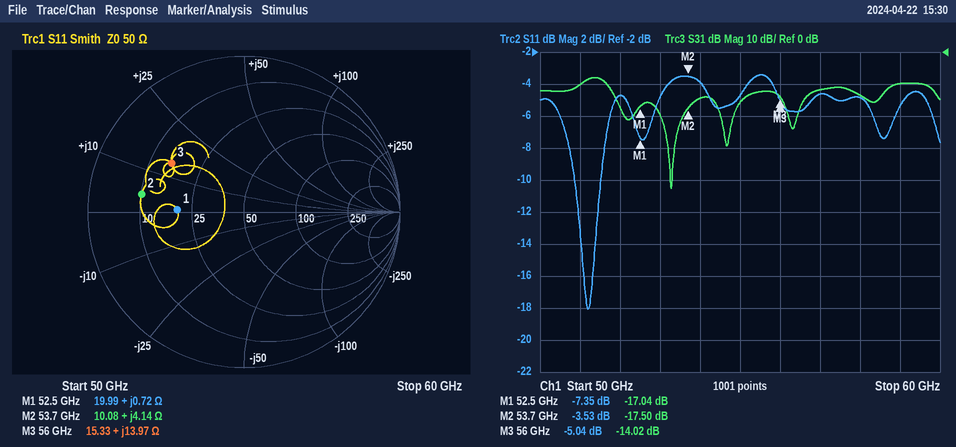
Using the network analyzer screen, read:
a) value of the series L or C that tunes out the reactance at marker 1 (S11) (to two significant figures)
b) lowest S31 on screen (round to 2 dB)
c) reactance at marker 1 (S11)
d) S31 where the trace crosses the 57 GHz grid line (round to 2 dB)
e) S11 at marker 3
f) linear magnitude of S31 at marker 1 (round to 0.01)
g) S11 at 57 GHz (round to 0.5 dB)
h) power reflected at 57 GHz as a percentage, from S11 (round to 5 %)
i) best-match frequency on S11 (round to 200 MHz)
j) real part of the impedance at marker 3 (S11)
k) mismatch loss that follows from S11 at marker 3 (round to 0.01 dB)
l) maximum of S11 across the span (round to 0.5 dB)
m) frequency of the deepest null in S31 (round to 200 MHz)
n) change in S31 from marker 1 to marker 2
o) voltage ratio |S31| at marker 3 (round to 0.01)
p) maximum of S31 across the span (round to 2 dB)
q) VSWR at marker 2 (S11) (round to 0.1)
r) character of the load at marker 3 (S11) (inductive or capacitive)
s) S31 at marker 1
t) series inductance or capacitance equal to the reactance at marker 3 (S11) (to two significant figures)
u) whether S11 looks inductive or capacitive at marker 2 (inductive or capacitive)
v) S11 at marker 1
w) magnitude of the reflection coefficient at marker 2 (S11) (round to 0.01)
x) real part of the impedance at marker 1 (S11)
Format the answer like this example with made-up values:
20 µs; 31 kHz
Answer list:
4.2 pF; -42 dB; +0.72 Ω; -12 dB; -5.04 dB; 0.14; -4.5 dB; 35 %; 51.2 GHz; 15.33 Ω; 1.63 dB; -3.5 dB; 53.2 GHz; -0.46 dB; 0.20; -8 dB; 5.0; inductive; -17.04 dB; 40 pH; inductive; -7.35 dB; 0.67; 19.99 Ω
